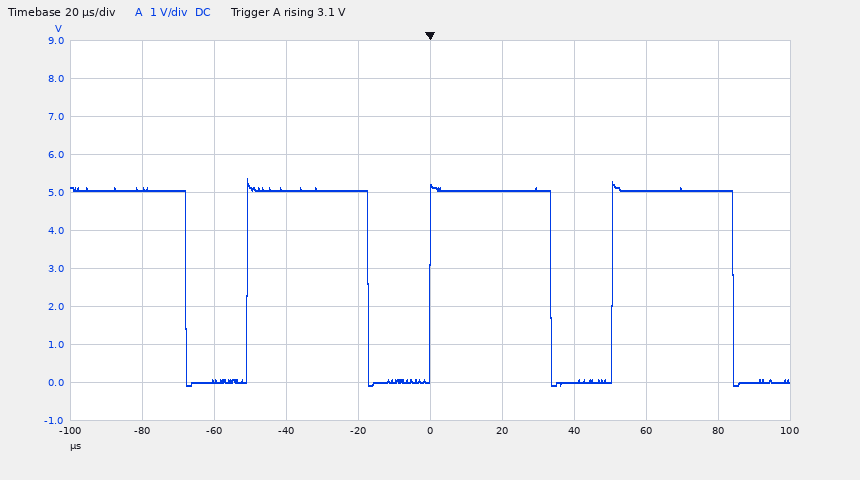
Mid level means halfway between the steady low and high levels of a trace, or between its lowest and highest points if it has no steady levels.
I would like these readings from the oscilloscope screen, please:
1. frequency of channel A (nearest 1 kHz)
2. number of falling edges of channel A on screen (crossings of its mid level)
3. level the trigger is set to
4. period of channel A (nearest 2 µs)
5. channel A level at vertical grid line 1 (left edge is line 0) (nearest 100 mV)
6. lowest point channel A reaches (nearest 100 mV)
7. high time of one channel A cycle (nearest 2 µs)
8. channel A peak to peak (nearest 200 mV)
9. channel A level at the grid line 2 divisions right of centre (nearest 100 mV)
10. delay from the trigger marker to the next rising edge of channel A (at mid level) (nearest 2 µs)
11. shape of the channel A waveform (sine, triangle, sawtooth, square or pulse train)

20 kHz
4
3.1 V
50 µs
5.1 V
-100 mV
34 µs
5.4 V
0.0 V
50 µs
pulse train
